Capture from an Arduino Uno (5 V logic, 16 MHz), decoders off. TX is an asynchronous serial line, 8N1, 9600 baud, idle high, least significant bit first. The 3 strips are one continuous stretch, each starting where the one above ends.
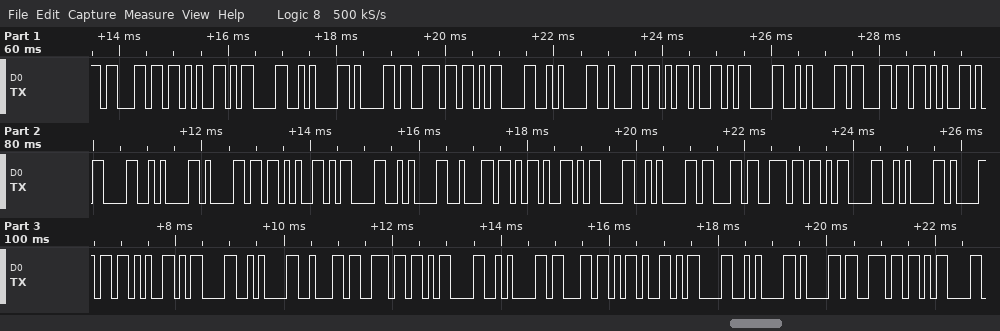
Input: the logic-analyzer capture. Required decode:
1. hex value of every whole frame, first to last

63 2B 0D 0A 61 6E 0D 0A 62 2D 0D 0A 63 2B 0D 0A 61 2B 0D 0A 62 2D 0D 0A 63 6E 0D 0A 61 2B 0D 0A 62 6E 0D 0A 63 2D 0D 0A 61 6E 0D
